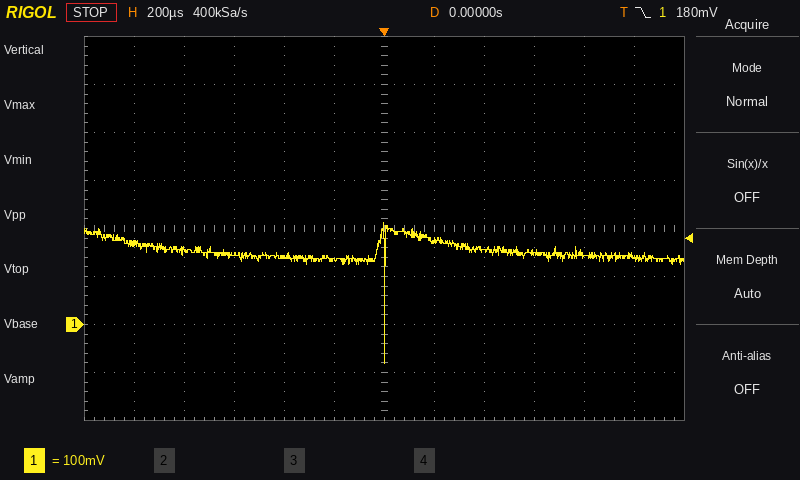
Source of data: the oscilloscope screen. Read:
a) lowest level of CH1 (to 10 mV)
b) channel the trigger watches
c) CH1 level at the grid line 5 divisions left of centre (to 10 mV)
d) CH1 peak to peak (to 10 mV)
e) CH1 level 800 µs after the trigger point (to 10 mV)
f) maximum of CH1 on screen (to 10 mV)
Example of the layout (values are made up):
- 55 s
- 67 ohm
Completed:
- -80 mV
- CH1
- 170 mV
- 290 mV
- 140 mV
- 210 mV
